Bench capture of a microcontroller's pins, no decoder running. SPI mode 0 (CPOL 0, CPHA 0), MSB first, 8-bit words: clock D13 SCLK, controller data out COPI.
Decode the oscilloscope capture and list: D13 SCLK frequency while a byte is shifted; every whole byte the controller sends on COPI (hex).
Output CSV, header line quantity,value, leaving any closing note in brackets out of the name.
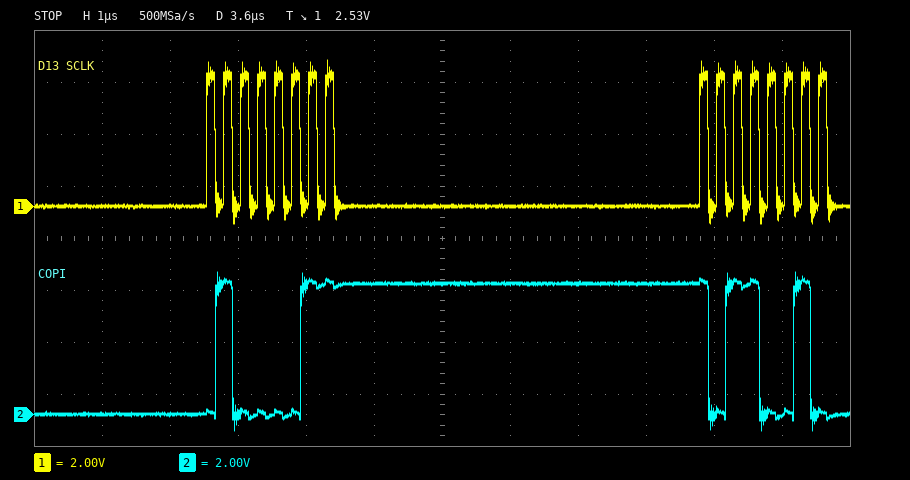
quantity,value
D13 SCLK frequency while a byte is shifted,4 MHz
every whole byte the controller sends on COPI,43 B2
